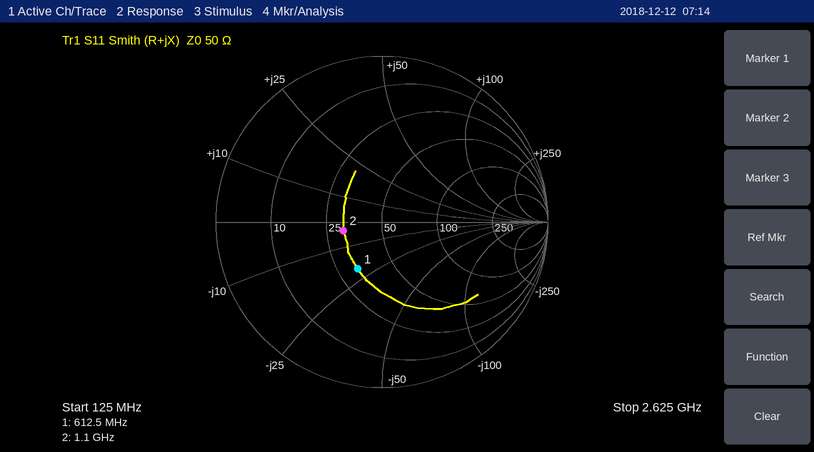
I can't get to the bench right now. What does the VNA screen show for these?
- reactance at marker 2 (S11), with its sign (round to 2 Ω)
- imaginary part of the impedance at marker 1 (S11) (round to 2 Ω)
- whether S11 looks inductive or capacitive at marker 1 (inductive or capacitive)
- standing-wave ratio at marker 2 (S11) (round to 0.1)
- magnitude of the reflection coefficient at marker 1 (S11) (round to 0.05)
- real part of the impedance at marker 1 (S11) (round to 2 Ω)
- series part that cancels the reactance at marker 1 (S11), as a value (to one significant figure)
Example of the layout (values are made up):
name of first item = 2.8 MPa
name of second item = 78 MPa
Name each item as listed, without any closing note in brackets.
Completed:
reactance at marker 2 (S11), with its sign = -4 Ω
imaginary part of the impedance at marker 1 (S11) = -20 Ω
whether S11 looks inductive or capacitive at marker 1 = capacitive
standing-wave ratio at marker 2 (S11) = 1.6
magnitude of the reflection coefficient at marker 1 (S11) = 0.30
real part of the impedance at marker 1 (S11) = 32 Ω
series part that cancels the reactance at marker 1 (S11), as a value = 5 nH
